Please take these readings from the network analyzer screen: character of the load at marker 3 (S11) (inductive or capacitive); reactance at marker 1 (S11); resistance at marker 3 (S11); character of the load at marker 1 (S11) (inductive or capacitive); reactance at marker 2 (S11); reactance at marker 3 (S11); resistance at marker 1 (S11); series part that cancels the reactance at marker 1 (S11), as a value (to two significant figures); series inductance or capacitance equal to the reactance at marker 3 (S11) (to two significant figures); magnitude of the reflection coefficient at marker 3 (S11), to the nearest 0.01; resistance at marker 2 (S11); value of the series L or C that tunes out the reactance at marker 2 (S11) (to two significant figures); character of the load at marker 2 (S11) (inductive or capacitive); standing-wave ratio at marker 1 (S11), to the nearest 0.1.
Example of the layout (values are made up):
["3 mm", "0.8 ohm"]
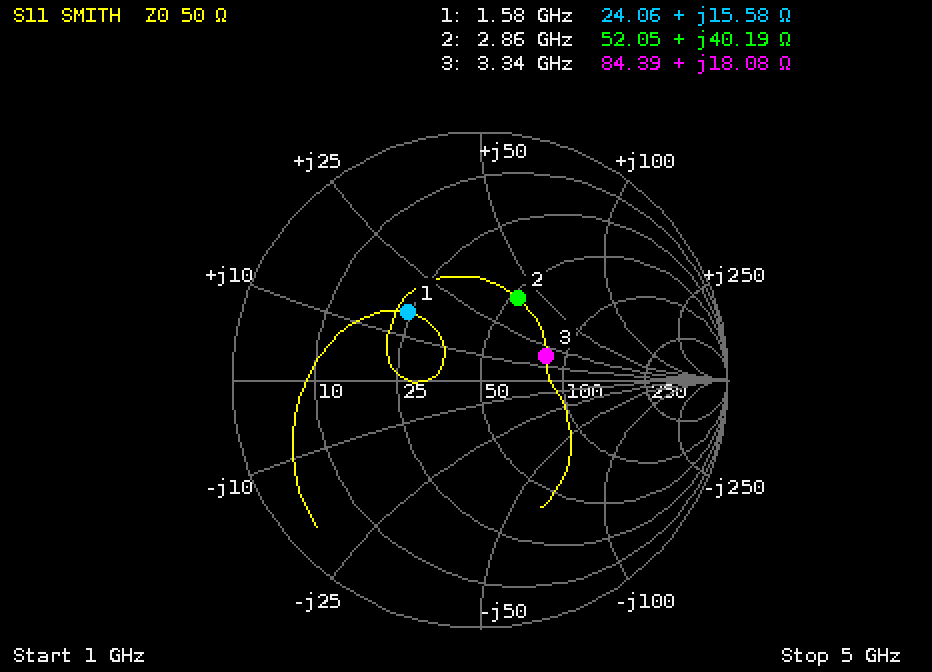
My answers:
["inductive", "+15.58 Ω", "84.39 Ω", "inductive", "+40.19 Ω", "+18.08 Ω", "24.06 Ω", "6.5 pF", "860 pH", "0.29", "52.05 Ω", "1.4 pF", "inductive", "2.3"]
